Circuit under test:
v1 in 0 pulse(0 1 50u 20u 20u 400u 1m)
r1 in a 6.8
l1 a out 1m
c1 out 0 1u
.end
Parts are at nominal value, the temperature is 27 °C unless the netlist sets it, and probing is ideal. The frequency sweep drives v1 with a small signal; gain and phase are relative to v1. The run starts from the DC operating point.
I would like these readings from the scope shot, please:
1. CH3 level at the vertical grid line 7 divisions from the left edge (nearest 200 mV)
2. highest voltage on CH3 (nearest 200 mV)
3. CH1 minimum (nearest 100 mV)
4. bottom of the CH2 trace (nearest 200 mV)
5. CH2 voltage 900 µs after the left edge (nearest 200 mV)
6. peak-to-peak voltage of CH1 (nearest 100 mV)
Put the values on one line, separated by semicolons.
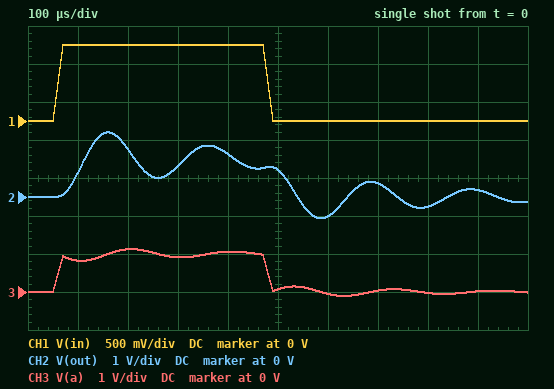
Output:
0 V; 1.2 V; 0 V; -600 mV; 200 mV; 1.0 V
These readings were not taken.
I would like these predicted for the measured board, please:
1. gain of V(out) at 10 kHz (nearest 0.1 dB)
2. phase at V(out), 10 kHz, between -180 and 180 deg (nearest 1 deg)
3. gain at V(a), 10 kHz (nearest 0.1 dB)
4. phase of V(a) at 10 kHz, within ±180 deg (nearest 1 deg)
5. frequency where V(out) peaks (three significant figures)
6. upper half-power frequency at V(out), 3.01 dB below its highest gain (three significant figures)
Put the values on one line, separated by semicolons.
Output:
-9.5 dB; -172 deg; -0.1 dB; 8 deg; 4.97 kHz; 5.49 kHz
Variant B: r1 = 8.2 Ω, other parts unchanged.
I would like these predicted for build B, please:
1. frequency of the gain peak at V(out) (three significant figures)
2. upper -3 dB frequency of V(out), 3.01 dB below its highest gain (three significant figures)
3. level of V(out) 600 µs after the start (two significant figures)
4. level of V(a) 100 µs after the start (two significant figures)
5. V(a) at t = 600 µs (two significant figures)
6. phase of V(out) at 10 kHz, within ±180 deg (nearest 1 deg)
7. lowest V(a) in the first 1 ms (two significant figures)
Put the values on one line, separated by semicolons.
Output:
4.95 kHz; 5.57 kHz; -490 mV; 790 mV; -65 mV; -170 deg; -120 mV
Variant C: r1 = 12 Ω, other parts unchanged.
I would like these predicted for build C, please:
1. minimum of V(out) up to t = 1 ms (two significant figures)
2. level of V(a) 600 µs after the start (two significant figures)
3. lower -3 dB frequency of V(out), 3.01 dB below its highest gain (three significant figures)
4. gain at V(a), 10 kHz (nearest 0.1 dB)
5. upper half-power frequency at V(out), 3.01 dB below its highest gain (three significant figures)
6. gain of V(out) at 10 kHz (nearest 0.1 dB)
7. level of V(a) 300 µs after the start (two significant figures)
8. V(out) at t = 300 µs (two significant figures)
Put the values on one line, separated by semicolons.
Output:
-490 mV; -88 mV; 3.75 kHz; -0.3 dB; 5.74 kHz; -9.7 dB; 920 mV; 870 mV
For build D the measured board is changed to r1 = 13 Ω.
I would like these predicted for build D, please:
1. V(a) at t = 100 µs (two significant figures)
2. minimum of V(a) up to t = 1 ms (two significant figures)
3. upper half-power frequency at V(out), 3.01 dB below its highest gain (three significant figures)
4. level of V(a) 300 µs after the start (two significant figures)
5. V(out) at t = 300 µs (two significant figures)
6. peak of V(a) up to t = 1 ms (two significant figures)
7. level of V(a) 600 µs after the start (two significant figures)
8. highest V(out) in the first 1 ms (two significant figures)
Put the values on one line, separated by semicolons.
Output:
700 mV; -150 mV; 5.78 kHz; 920 mV; 870 mV; 1.2 V; -91 mV; 1.5 V
